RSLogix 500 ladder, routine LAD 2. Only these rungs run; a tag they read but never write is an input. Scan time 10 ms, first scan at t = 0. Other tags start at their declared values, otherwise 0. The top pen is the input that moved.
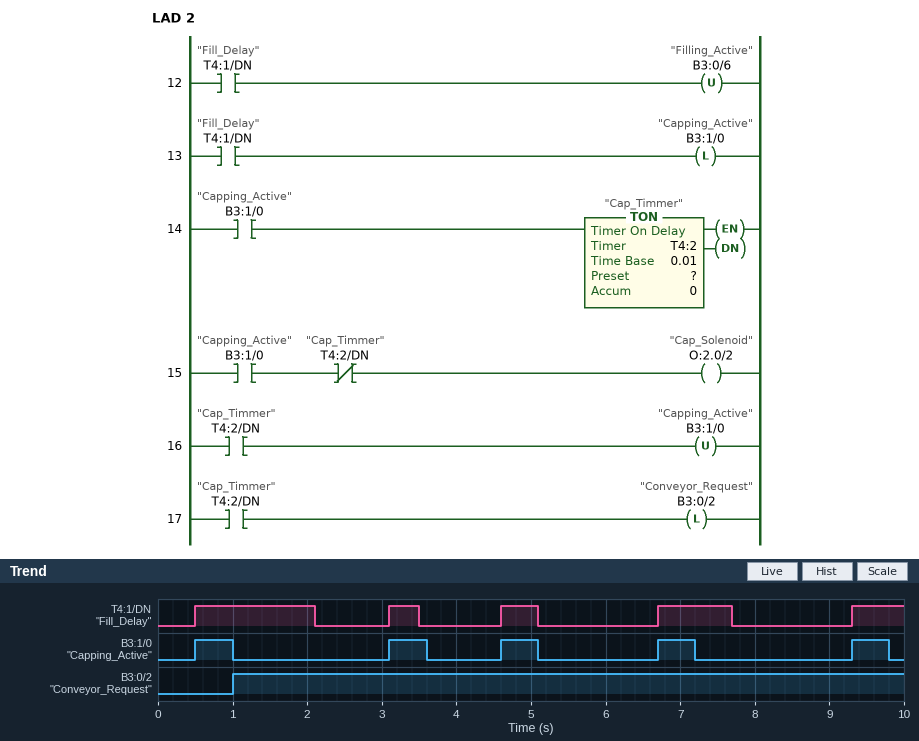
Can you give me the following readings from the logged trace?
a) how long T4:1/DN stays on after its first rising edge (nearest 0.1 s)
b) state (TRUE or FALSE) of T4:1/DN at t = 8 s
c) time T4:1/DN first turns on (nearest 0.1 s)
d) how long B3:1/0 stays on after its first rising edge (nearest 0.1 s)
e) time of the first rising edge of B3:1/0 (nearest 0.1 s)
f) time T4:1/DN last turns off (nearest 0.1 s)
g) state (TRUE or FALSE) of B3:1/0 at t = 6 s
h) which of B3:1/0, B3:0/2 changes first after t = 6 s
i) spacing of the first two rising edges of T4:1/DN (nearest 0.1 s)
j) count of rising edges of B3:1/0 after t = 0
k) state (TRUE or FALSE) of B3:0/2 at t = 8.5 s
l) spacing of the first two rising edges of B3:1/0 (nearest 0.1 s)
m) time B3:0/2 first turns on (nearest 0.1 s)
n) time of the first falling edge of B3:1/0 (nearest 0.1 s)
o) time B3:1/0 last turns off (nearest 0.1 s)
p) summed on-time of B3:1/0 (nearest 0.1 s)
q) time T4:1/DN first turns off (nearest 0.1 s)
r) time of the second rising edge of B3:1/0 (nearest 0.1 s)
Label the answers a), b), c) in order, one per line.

a) 1.6 s
b) FALSE
c) 0.5 s
d) 0.5 s
e) 0.5 s
f) 7.7 s
g) FALSE
h) B3:1/0
i) 2.6 s
j) 5
k) TRUE
l) 2.6 s
m) 1.0 s
n) 1.0 s
o) 9.8 s
p) 2.5 s
q) 2.1 s
r) 3.1 s
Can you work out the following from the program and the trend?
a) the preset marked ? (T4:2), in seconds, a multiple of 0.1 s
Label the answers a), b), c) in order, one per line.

a) 0.5 s
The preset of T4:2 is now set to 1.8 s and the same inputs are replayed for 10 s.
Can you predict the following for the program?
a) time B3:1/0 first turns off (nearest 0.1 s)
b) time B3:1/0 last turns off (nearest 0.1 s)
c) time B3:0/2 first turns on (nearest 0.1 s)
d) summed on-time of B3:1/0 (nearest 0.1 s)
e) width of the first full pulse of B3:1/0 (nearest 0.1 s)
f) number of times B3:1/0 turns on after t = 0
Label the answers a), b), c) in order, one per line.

a) 2.3 s
b) 8.5 s
c) 2.3 s
d) 6.1 s
e) 1.8 s
f) 4
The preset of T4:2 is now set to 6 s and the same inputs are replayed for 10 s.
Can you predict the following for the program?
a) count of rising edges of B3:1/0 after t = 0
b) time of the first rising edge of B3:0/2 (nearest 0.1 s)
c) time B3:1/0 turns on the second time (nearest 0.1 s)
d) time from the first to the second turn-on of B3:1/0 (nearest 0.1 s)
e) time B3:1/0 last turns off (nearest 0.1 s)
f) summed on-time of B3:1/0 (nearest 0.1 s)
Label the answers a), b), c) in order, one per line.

a) 2
b) 6.5 s
c) 6.7 s
d) 6.2 s
e) 6.5 s
f) 9.3 s
